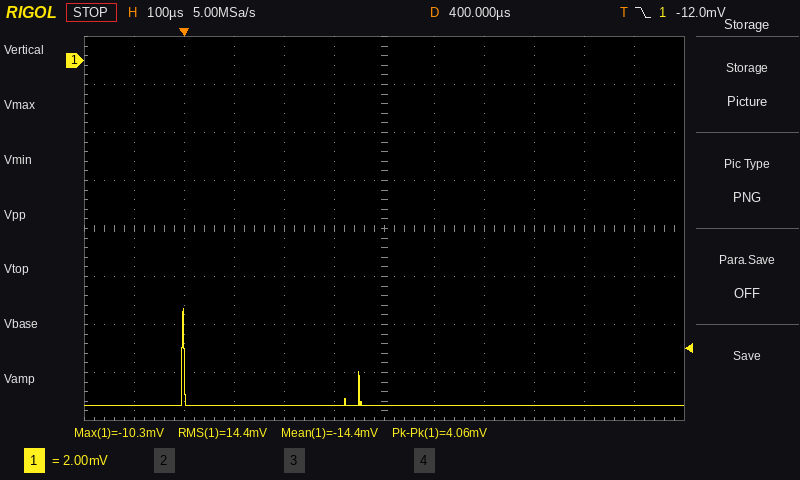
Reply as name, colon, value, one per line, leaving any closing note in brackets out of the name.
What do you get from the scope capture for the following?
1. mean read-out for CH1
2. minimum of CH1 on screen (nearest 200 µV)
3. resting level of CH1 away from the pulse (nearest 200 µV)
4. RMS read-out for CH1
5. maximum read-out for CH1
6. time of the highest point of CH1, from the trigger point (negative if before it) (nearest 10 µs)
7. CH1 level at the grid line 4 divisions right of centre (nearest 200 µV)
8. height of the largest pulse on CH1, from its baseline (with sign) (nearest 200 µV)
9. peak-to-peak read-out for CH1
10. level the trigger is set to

mean read-out for CH1: -14.4 mV
minimum of CH1 on screen: -14.4 mV
resting level of CH1 away from the pulse: -14.4 mV
RMS read-out for CH1: 14.4 mV
maximum read-out for CH1: -10.3 mV
time of the highest point of CH1, from the trigger point (negative if before it): 0 µs
CH1 level at the grid line 4 divisions right of centre: -14.4 mV
height of the largest pulse on CH1, from its baseline (with sign): +4.0 mV
peak-to-peak read-out for CH1: 4.06 mV
level the trigger is set to: -12.0 mV
